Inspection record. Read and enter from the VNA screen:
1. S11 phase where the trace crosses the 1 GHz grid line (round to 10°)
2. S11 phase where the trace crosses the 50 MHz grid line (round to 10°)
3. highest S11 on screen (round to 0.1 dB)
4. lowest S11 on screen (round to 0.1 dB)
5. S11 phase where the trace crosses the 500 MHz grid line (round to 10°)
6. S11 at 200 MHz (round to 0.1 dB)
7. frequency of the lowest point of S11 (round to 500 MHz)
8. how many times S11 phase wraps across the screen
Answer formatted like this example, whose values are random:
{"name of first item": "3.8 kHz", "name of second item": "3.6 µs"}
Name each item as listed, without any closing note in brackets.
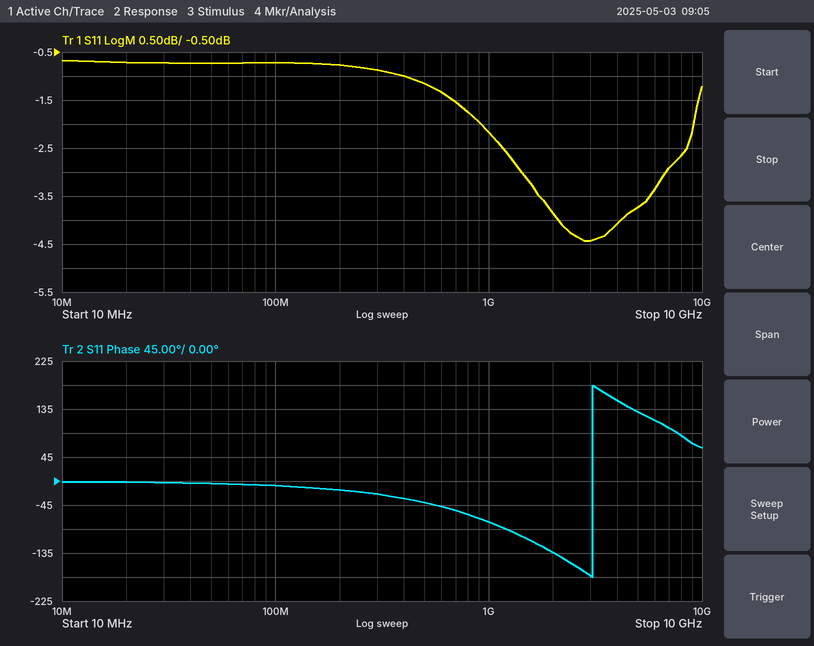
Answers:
{"S11 phase where the trace crosses the 1 GHz grid line": "-80°", "S11 phase where the trace crosses the 50 MHz grid line": "0°", "highest S11 on screen": "-0.7 dB", "lowest S11 on screen": "-4.4 dB", "S11 phase where the trace crosses the 500 MHz grid line": "-40°", "S11 at 200 MHz": "-0.8 dB", "frequency of the lowest point of S11": "3.0 GHz", "how many times S11 phase wraps across the screen": "1"}
